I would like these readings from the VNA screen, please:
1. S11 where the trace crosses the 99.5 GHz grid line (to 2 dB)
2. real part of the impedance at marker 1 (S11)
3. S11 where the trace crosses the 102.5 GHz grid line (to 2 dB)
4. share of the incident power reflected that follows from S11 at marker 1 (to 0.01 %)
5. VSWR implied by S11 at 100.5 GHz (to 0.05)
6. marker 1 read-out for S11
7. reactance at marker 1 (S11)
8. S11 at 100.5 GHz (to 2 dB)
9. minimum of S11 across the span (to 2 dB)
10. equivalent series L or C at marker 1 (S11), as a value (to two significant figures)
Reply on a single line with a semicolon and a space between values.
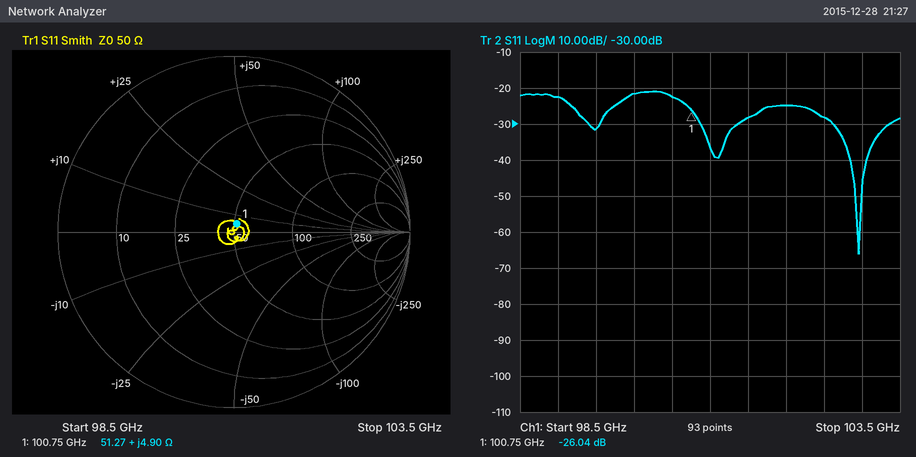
-32 dB; 51.27 Ω; -28 dB; 0.25 %; 1.15; -26.04 dB; +4.90 Ω; -22 dB; -66 dB; 7.7 pH
